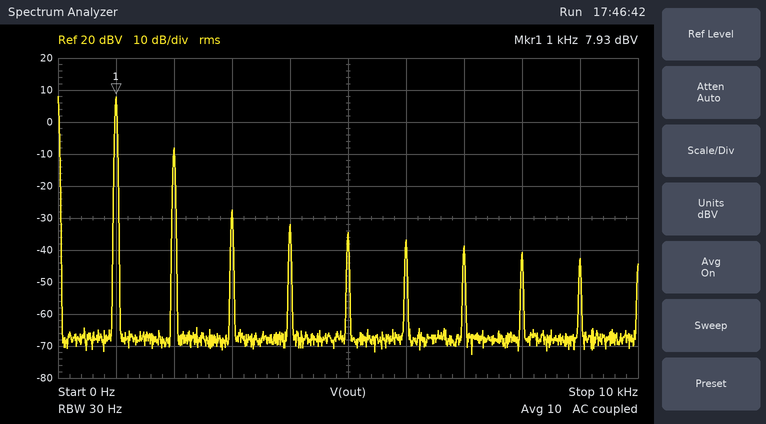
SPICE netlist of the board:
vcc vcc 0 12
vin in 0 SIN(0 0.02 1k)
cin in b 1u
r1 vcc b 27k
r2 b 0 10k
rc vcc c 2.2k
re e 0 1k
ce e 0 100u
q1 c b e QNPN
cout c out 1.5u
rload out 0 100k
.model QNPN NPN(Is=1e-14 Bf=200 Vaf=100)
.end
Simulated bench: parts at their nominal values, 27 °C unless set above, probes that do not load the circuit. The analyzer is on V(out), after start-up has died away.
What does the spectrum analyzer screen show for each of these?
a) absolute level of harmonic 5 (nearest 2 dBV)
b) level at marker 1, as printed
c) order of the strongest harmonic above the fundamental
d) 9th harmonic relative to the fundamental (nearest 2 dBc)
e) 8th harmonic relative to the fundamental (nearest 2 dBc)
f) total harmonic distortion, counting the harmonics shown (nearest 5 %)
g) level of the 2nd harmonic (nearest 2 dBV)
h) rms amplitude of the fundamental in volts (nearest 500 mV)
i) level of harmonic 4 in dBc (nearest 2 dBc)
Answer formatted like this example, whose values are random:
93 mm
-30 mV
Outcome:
-34 dBV
7.93 dBV
2
-50 dBc
-48 dBc
15 %
-8 dBV
2.5 V
-40 dBc
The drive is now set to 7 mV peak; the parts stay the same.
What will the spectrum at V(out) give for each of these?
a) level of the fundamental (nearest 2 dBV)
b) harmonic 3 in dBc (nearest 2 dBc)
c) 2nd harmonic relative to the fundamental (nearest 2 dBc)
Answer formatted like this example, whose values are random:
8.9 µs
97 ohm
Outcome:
0 dBV
-54 dBc
-24 dBc
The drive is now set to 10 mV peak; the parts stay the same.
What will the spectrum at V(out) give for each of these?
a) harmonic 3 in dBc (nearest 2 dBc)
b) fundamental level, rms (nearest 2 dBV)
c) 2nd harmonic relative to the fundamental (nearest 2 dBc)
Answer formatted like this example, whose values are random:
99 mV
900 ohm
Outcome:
-48 dBc
2 dBV
-22 dBc
